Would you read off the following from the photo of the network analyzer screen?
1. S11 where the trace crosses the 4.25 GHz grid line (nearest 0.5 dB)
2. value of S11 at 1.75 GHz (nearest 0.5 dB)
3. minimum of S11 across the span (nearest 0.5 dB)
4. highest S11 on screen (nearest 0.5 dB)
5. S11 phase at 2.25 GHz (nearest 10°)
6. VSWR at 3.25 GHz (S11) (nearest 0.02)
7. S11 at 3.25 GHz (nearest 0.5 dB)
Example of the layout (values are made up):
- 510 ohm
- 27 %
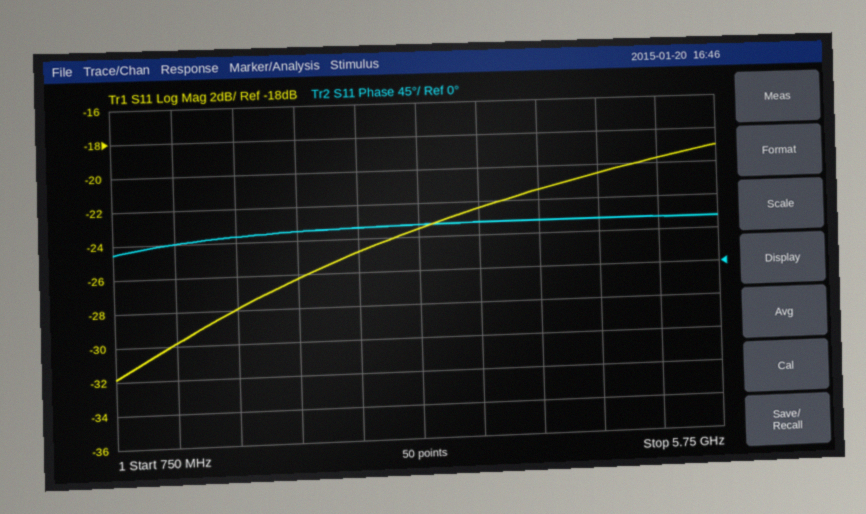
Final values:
- -21.5 dB
- -28.0 dB
- -32.0 dB
- -19.0 dB
- 60°
- 1.14
- -23.5 dB
